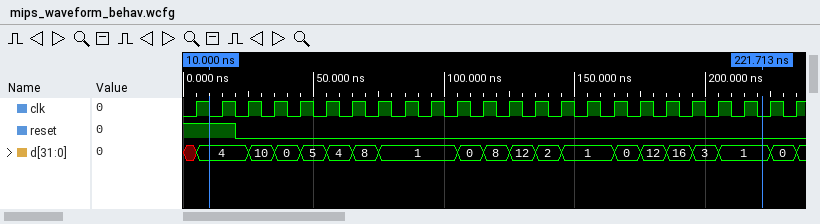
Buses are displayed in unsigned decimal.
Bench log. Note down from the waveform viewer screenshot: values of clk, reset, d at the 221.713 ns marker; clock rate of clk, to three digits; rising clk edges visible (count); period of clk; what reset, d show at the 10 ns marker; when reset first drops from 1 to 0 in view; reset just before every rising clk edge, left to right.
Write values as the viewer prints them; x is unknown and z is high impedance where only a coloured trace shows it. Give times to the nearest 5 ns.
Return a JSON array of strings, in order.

["clk=0, reset=0, d=1", "100 MHz", "24", "10 ns", "reset=1, d=4", "20 ns", "1 1 0 0 0 0 0 0 0 0 0 0 0 0 0 0 0 0 0 0 0 0 0 0"]
